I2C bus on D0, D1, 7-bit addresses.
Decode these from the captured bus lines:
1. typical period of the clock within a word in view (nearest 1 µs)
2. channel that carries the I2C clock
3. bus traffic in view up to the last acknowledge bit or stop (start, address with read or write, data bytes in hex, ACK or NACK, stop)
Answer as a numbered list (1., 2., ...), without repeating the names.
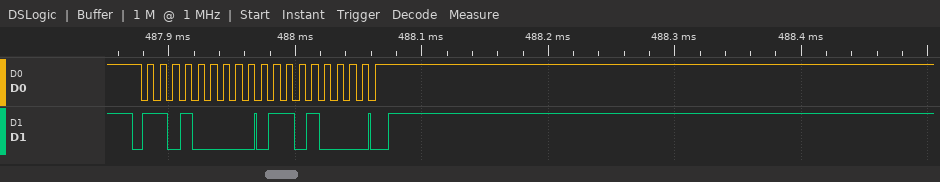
1. 10 µs
2. D0
3. start, address 68 write ACK, 68 ACK, stop
